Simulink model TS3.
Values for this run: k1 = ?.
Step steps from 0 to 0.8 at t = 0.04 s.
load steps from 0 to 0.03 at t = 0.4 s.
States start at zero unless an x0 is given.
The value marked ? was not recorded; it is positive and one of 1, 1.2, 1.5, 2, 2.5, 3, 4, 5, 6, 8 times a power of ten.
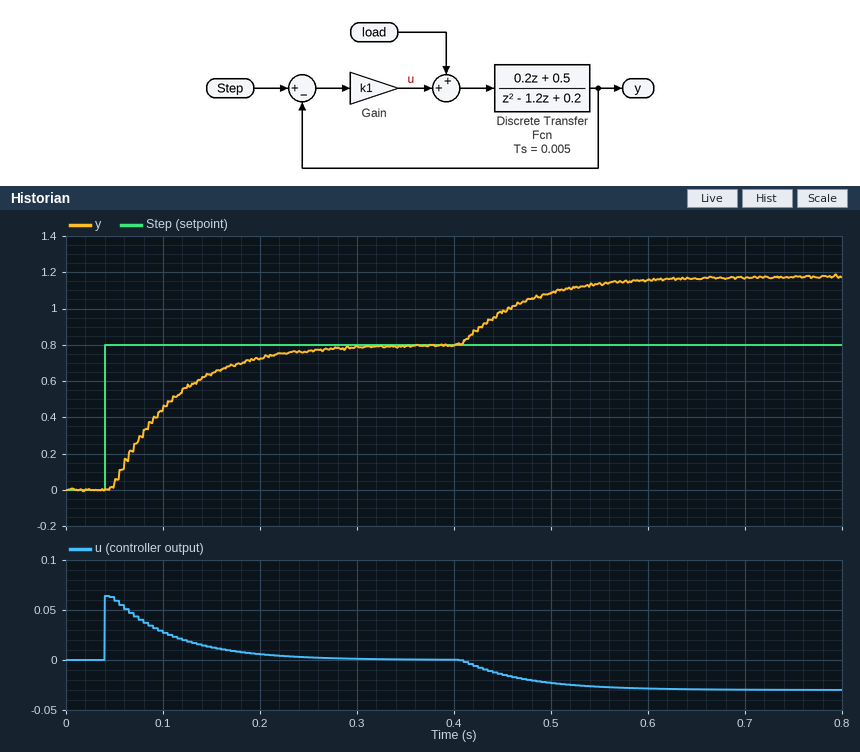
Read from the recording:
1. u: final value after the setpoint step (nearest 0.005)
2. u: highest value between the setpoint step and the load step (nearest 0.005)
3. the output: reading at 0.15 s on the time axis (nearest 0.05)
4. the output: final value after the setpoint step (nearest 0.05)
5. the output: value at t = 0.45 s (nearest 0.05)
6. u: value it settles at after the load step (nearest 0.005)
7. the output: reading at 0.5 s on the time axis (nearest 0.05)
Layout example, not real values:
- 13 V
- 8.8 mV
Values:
- 0.000
- 0.065
- 0.65
- 0.80
- 1.00
- -0.030
- 1.10
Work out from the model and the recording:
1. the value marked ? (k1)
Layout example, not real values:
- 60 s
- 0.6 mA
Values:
- 0.08
